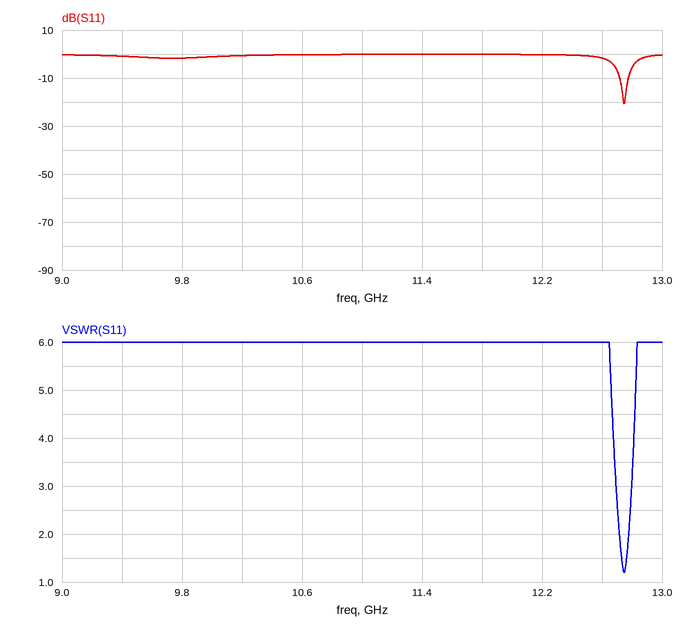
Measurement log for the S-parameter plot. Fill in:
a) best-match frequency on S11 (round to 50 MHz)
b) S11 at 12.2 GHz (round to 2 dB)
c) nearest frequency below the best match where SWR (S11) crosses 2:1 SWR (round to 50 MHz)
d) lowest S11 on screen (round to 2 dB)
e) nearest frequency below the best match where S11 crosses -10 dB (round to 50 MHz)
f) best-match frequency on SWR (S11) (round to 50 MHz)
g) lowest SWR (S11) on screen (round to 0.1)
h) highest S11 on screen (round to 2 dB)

12.75 GHz
0 dB
12.70 GHz
-20 dB
12.70 GHz
12.75 GHz
1.2
0 dB
